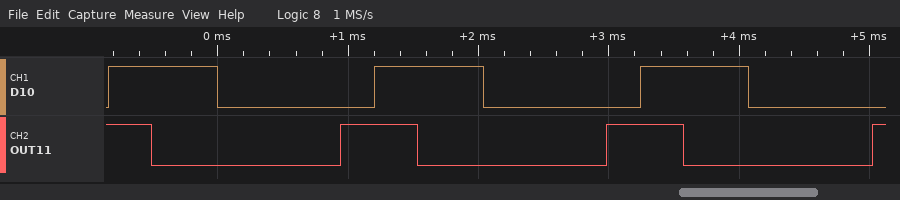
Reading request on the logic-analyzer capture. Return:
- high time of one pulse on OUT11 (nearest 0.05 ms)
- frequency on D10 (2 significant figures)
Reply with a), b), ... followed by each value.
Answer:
a) 0.60 ms
b) 490 Hz
